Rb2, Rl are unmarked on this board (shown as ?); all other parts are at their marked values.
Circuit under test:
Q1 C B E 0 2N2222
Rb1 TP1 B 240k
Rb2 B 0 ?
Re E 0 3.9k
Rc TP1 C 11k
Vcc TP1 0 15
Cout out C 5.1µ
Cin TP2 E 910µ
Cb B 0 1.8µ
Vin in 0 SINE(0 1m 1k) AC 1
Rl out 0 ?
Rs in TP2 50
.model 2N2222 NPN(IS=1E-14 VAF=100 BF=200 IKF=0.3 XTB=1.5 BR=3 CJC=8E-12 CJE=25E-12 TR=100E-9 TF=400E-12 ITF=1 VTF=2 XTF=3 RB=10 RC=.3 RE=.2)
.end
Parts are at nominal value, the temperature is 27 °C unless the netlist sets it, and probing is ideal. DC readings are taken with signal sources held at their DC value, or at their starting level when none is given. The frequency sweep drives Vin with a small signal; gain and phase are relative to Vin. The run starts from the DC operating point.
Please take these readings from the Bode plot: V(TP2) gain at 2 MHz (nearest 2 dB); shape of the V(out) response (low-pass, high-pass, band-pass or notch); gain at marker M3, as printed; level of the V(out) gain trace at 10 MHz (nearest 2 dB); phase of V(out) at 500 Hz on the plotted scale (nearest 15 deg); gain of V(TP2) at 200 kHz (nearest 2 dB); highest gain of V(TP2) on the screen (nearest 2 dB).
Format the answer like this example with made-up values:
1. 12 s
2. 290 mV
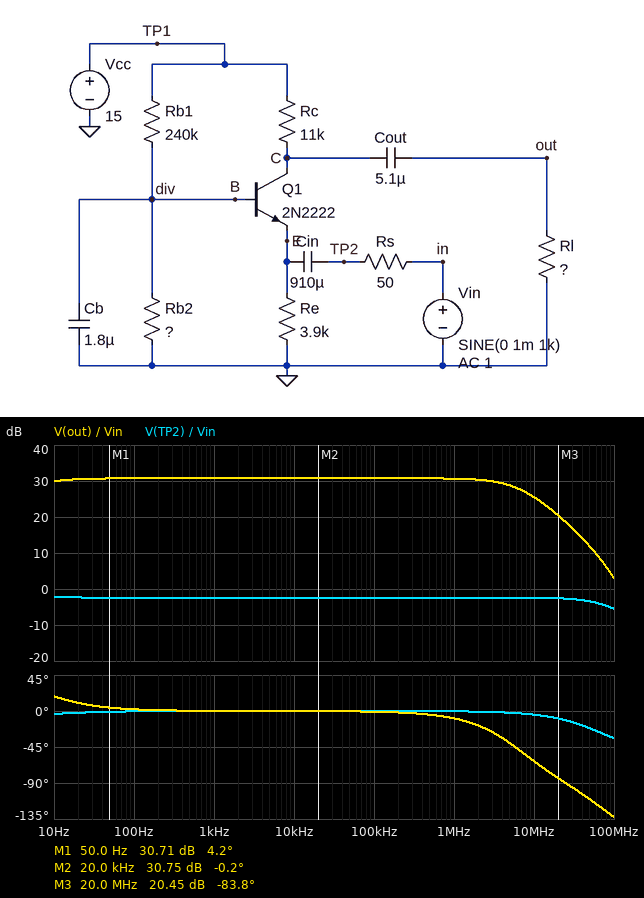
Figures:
1. -2 dB
2. low-pass
3. 20.45 dB
4. 26 dB
5. 0 deg
6. -2 dB
7. -2 dB
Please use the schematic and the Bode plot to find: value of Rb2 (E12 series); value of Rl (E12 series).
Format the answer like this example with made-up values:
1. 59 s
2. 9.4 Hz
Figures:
1. 22 kΩ
2. 22 kΩ
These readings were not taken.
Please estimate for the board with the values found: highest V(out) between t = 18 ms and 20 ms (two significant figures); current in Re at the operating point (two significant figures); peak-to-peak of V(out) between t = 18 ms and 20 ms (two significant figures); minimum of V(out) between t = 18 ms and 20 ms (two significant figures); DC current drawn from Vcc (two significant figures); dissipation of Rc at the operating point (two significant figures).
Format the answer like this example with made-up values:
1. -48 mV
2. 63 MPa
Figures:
1. 34 mV
2. 160 µA
3. 69 mV
4. -35 mV
5. 220 µA
6. 290 µW
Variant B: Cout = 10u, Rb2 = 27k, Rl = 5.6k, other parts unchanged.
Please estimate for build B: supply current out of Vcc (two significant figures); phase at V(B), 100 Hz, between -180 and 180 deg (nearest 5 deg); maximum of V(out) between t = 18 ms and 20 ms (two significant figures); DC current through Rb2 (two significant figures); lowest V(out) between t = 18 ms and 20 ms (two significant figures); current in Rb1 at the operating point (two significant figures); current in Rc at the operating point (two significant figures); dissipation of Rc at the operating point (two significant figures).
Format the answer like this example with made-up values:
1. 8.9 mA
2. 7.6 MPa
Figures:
1. 280 µA
2. -85 deg
3. 22 mV
4. 55 µA
5. -22 mV
6. 56 µA
7. 220 µA
8. 550 µW
